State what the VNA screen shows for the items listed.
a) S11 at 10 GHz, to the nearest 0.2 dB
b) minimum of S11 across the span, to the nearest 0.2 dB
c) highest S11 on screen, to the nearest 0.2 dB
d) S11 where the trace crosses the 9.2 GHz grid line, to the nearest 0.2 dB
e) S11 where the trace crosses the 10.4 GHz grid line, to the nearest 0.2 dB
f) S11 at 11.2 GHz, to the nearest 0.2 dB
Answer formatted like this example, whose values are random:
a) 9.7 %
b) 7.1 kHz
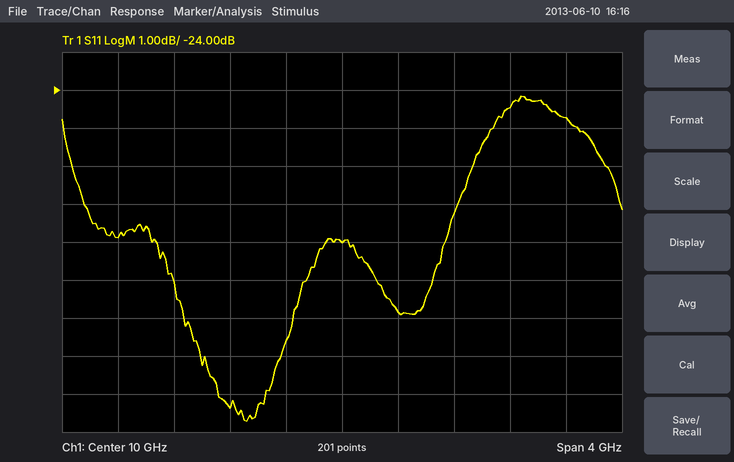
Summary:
a) -28.0 dB
b) -32.8 dB
c) -24.2 dB
d) -32.4 dB
e) -29.8 dB
f) -24.4 dB
